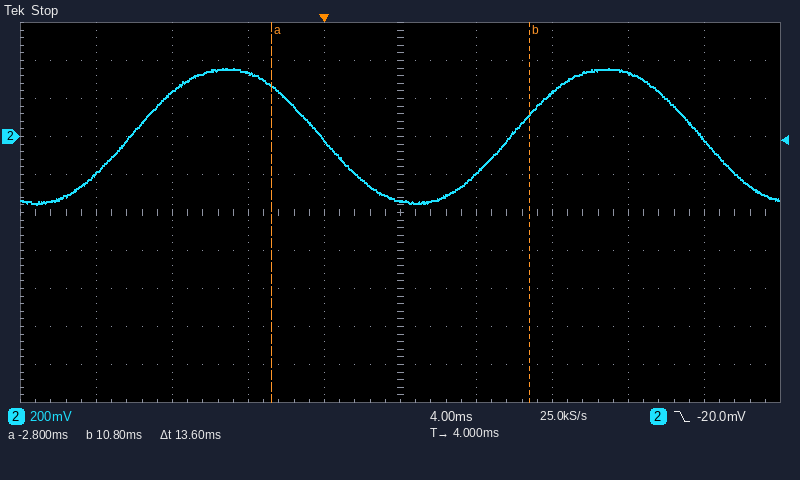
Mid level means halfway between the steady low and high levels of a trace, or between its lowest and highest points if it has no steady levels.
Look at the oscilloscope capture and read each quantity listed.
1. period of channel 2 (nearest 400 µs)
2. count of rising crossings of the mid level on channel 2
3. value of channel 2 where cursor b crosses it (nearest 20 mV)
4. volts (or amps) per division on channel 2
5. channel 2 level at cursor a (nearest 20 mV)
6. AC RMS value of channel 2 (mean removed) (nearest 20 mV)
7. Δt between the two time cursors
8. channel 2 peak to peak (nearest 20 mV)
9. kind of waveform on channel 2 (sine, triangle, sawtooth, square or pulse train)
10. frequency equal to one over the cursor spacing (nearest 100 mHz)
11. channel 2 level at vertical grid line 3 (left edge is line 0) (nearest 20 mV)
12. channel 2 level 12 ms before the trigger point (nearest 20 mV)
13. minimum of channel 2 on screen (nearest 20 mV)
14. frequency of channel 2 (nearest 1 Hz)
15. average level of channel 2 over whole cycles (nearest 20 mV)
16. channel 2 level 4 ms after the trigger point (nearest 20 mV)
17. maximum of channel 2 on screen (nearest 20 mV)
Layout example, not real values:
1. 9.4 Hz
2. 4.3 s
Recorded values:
1. 20.0 ms
2. 2
3. 120 mV
4. 200 mV
5. 260 mV
6. 260 mV
7. 13.6 ms
8. 720 mV
9. sine
10. 73.5 Hz
11. 340 mV
12. -200 mV
13. -360 mV
14. 50 Hz
15. 0 mV
16. -340 mV
17. 360 mV
